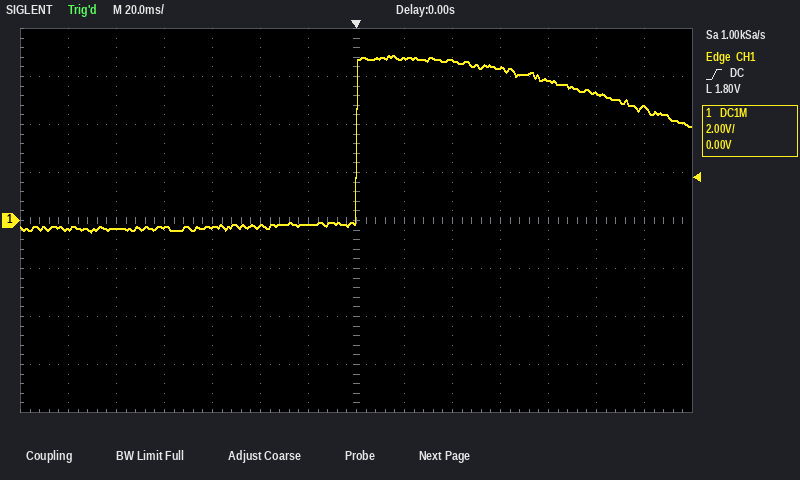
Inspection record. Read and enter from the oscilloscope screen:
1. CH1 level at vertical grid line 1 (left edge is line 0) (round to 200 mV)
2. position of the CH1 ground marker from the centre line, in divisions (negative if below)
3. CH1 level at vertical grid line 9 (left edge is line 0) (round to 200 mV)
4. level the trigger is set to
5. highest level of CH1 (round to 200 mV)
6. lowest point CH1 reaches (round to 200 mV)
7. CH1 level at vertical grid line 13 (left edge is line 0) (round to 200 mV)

-400 mV
0.0 div
6.6 V
1.80 V
6.8 V
-400 mV
4.8 V
